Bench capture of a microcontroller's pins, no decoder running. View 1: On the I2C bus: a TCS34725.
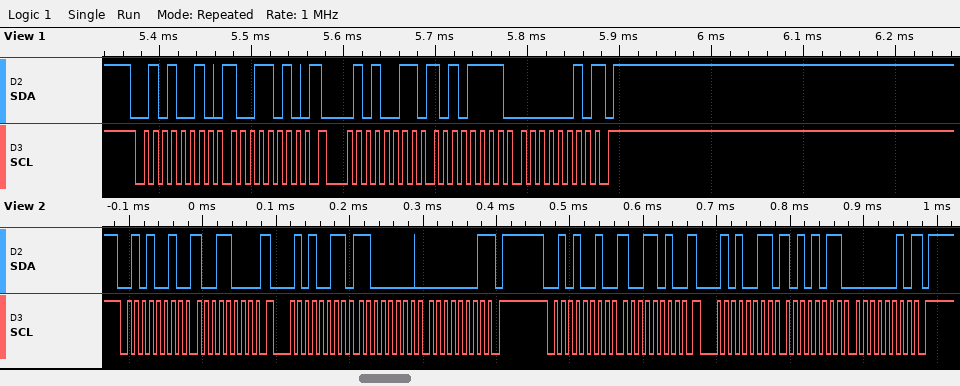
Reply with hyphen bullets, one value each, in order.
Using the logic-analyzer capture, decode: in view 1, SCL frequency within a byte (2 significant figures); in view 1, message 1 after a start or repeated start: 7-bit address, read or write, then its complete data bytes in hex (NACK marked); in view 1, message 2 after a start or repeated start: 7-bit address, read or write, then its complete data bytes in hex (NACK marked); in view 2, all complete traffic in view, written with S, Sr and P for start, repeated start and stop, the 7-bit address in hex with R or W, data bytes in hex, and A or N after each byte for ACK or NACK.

- 100 kHz
- 0x29 write: 9A
- 0x29 read: AF 02 NACK
- S 29W A 98 A Sr 29R A C0 A 01 N P S 29W A 9A A Sr 29R A AB A 02 N P
